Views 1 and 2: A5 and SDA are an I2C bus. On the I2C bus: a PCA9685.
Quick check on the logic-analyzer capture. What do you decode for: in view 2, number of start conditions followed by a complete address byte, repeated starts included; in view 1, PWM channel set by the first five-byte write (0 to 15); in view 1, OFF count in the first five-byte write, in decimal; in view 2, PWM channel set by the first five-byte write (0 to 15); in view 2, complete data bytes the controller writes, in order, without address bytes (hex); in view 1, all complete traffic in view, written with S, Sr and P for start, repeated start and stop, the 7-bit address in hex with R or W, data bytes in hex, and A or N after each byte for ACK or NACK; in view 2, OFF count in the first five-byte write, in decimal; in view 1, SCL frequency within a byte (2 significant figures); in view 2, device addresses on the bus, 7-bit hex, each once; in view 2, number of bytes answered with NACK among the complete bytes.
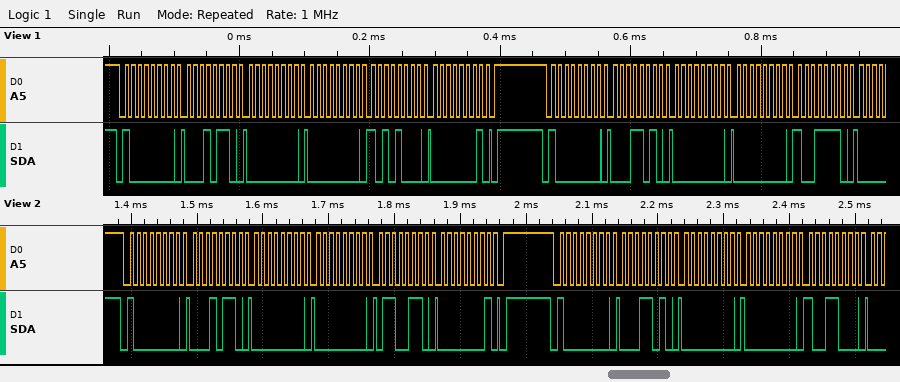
2
4
424
4
16 00 00 66 01 1A 00 00 98
S 40W A 16 A 00 A 00 A A8 A 01 A P S 40W A 1A A 00 A 00 A 9E A
358
100 kHz
0x40
0
